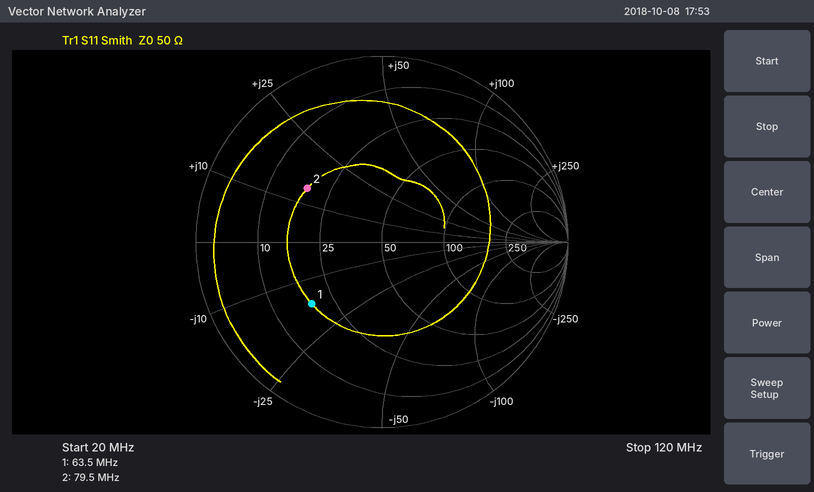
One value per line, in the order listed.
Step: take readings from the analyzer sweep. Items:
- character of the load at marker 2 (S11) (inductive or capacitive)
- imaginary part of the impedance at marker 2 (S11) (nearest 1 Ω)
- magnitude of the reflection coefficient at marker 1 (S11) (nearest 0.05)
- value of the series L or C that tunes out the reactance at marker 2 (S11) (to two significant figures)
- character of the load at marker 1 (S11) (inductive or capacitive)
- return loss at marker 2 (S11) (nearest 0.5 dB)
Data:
inductive
+14 Ω
0.50
140 pF
capacitive
6.0 dB
